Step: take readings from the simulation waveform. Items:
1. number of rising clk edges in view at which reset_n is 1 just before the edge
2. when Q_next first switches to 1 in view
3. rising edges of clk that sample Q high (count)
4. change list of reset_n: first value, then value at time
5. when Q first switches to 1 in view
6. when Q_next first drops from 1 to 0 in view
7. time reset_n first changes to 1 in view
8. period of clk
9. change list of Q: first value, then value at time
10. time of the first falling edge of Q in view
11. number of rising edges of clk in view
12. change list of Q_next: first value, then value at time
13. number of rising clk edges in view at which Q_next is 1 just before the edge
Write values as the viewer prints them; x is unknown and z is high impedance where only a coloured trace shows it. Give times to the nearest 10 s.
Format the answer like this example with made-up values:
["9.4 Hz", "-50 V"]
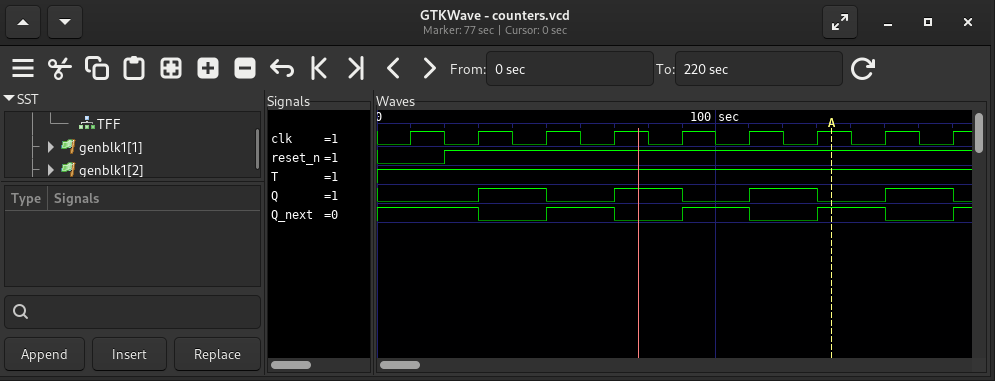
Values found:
["8", "50 s", "4", "0, 1 at 20 s", "30 s", "30 s", "20 s", "20 s", "0, 1 at 30 s, 0 at 50 s, 1 at 70 s, 0 at 90 s, 1 at 110 s, 0 at 130 s, 1 at 150 s, 0 at 170 s", "50 s", "9", "1, 0 at 30 s, 1 at 50 s, 0 at 70 s, 1 at 90 s, 0 at 110 s, 1 at 130 s, 0 at 150 s, 1 at 170 s", "5"]
